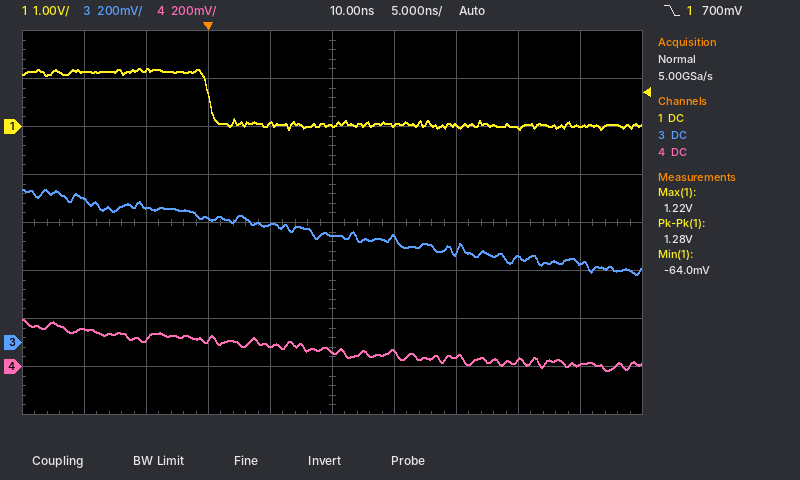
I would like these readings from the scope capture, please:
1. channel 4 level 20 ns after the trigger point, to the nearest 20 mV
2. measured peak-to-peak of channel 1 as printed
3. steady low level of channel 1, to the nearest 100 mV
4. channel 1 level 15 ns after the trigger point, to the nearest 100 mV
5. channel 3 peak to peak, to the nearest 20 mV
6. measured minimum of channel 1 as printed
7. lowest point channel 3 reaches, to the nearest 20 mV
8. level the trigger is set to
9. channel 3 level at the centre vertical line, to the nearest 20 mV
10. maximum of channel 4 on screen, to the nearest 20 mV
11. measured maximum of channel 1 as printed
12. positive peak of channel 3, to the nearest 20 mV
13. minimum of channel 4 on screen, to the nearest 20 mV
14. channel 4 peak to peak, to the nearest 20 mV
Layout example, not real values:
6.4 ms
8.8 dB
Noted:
40 mV
1.28 V
0.0 V
0.0 V
360 mV
-64.0 mV
280 mV
700 mV
440 mV
200 mV
1.22 V
640 mV
-20 mV
220 mV
